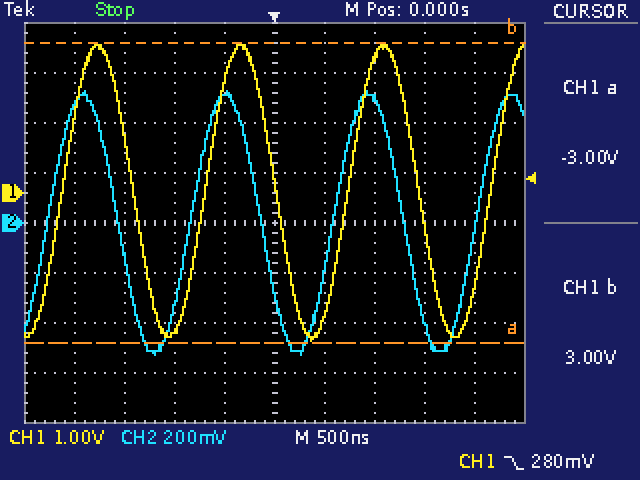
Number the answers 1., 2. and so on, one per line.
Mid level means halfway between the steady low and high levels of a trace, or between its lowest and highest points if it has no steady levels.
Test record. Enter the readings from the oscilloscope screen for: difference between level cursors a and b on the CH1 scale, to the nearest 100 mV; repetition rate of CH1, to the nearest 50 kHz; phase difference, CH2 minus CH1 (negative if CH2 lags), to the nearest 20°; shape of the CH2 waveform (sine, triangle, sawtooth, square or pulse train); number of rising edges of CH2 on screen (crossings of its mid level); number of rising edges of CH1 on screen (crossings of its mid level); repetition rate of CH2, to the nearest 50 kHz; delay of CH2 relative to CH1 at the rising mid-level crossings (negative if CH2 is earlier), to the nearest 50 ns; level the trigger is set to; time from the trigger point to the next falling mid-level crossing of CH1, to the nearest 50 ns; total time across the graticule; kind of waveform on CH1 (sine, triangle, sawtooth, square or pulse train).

1. 6.0 V
2. 700 kHz
3. +40°
4. sine
5. 4
6. 4
7. 700 kHz
8. -150 ns
9. 280 mV
10. 1.45 µs
11. 5 µs
12. sine
